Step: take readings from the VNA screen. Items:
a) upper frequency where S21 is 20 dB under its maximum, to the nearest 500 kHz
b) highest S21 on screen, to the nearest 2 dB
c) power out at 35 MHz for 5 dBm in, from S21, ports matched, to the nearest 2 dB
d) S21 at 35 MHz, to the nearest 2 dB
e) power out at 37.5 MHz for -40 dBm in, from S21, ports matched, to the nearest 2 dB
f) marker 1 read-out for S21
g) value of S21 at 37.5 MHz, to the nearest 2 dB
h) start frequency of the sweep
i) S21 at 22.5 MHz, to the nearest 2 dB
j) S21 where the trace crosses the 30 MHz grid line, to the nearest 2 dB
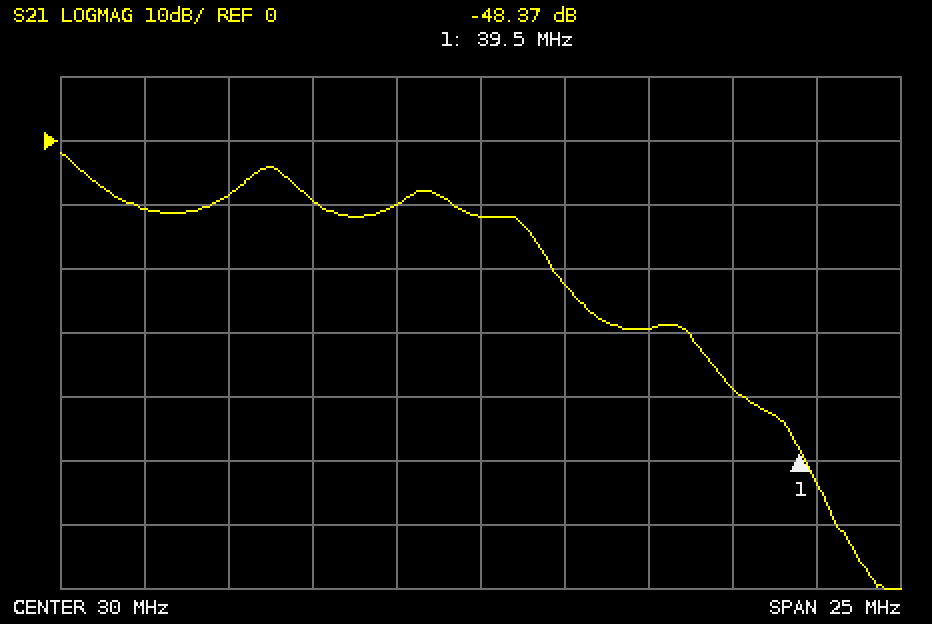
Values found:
32.5 MHz
-2 dB
-24 dBm
-30 dB
-78 dBm
-48.37 dB
-38 dB
17.5 MHz
-8 dB
-12 dB
